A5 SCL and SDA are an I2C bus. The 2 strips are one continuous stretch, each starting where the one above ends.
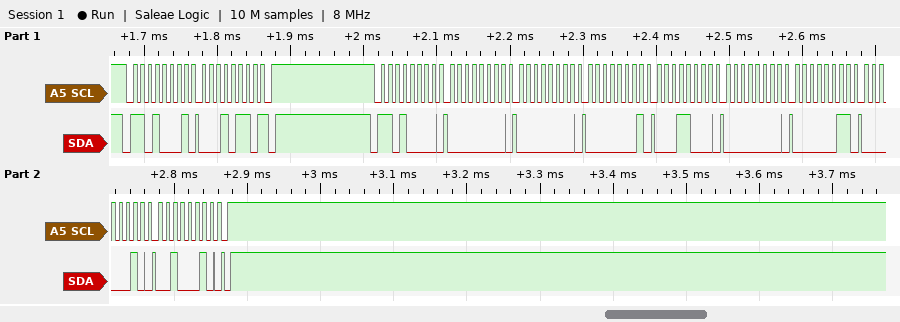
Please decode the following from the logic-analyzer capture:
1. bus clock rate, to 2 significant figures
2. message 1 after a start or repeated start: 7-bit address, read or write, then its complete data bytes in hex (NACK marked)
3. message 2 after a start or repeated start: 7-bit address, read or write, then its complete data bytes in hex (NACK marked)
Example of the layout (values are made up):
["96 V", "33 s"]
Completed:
["100 kHz", "0x68 read: 16 NACK", "0x68 write: 00 00 01 18 00 03 02 22"]
